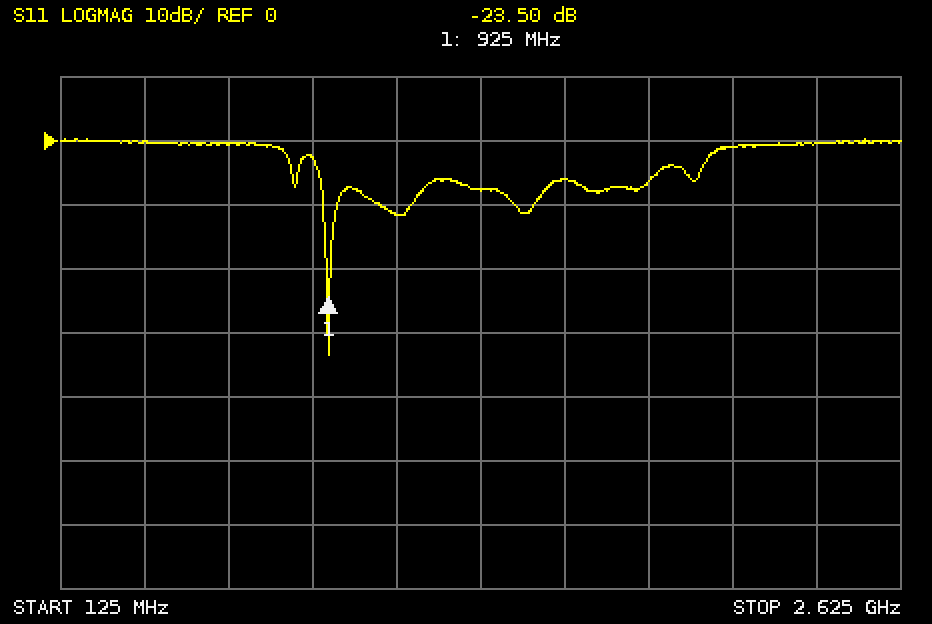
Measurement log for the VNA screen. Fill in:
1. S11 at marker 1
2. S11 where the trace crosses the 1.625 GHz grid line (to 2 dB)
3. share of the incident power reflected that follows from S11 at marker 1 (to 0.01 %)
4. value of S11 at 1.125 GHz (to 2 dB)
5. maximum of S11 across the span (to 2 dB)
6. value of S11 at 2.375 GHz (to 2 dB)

-23.50 dB
-6 dB
0.45 %
-12 dB
0 dB
0 dB
